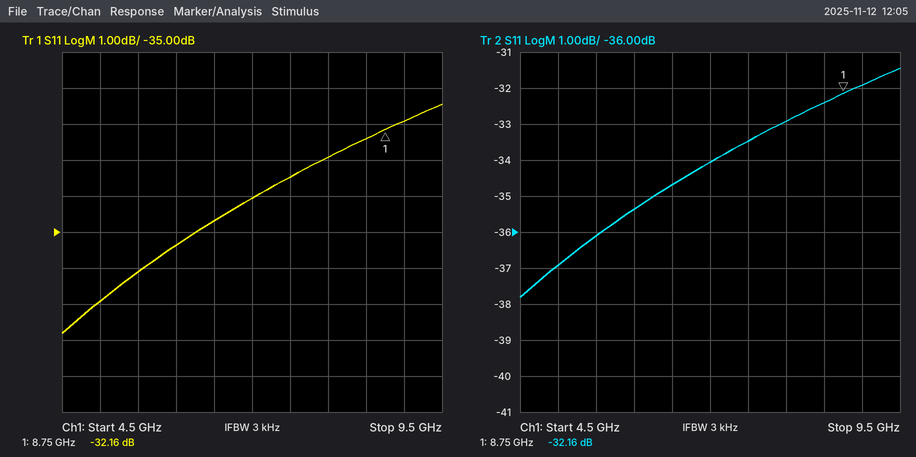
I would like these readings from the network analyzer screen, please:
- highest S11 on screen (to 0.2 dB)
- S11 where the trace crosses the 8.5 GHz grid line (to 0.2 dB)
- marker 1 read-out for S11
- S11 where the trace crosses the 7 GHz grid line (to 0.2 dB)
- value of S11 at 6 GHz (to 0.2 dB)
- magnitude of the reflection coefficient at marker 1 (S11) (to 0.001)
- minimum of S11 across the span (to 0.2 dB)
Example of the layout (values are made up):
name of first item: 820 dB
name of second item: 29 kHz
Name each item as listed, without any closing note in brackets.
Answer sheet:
highest S11 on screen: -31.4 dB
S11 where the trace crosses the 8.5 GHz grid line: -32.4 dB
marker 1 read-out for S11: -32.16 dB
S11 where the trace crosses the 7 GHz grid line: -34.0 dB
value of S11 at 6 GHz: -35.4 dB
magnitude of the reflection coefficient at marker 1 (S11): 0.025
minimum of S11 across the span: -37.8 dB
